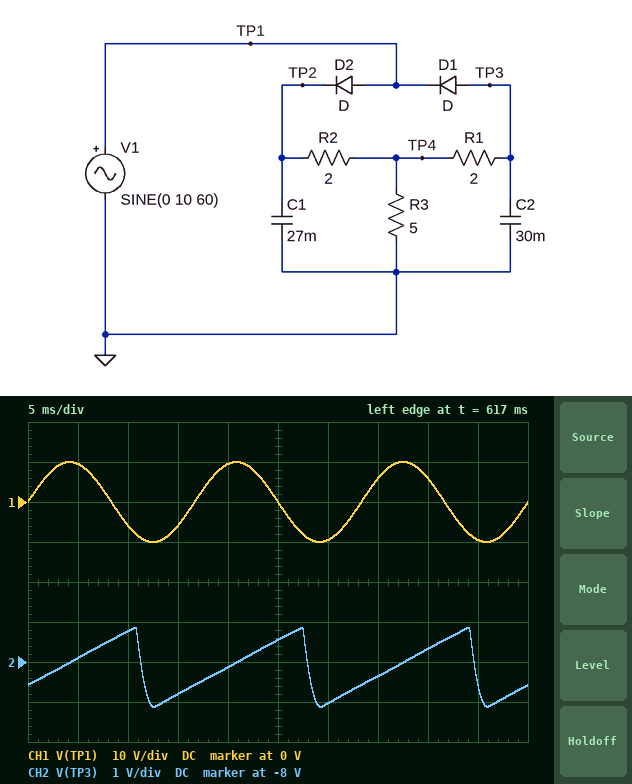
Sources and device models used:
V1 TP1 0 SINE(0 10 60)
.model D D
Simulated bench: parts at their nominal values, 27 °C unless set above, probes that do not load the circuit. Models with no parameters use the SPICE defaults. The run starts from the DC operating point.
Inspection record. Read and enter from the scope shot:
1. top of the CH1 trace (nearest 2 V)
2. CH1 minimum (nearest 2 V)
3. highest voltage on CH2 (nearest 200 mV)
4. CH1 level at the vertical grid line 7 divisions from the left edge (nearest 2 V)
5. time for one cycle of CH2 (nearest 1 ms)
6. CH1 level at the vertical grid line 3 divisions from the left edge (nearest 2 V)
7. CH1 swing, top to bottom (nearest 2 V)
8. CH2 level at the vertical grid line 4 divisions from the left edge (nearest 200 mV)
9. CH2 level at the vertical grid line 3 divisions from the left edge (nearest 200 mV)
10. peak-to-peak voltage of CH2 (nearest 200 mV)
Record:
10 V
-10 V
-7.2 V
6 V
17 ms
-6 V
20 V
-8.2 V
-8.8 V
2.0 V
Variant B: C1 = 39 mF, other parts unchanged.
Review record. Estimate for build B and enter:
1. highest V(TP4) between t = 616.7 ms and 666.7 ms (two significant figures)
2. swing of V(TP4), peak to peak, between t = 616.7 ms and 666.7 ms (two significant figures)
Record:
560 mV
920 mV
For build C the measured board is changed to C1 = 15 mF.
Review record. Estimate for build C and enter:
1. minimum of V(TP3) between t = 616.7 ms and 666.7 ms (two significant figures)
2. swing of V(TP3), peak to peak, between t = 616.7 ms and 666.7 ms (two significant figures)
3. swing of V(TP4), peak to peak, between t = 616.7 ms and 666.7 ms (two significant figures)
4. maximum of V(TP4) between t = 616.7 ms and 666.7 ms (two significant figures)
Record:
-9.1 V
1.9 V
1.6 V
450 mV
